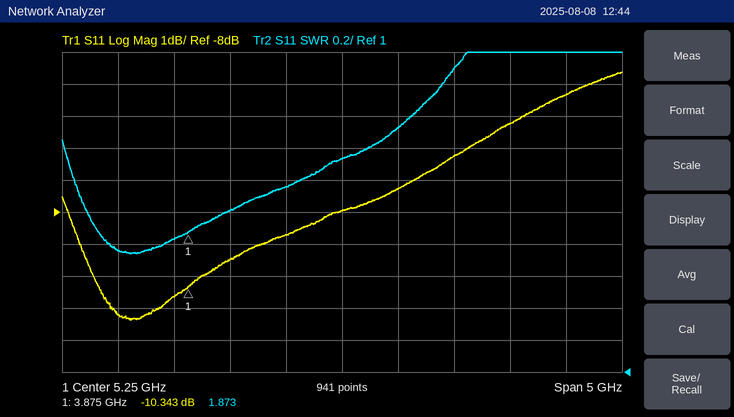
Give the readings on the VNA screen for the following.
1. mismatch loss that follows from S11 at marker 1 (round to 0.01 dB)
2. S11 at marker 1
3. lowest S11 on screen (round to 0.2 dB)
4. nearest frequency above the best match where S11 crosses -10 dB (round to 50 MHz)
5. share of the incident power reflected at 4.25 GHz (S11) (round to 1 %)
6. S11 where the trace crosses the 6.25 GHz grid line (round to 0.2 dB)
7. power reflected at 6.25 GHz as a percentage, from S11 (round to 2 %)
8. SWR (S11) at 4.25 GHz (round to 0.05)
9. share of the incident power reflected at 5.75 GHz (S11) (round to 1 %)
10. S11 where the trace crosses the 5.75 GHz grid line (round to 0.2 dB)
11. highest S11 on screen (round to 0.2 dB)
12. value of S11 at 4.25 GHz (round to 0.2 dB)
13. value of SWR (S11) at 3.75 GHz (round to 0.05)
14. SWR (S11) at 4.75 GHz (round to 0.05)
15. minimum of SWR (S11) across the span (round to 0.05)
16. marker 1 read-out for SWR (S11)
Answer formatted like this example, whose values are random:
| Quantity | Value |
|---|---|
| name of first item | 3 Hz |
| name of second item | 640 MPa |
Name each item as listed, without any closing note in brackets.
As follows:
| Quantity | Value |
|---|---|
| mismatch loss that follows from S11 at marker 1 | 0.42 dB |
| S11 at marker 1 | -10.343 dB |
| lowest S11 on screen | -11.4 dB |
| nearest frequency above the best match where S11 crosses -10 dB | 4.00 GHz |
| share of the incident power reflected at 4.25 GHz (S11) | 11 % |
| S11 where the trace crosses the 6.25 GHz grid line | -6.2 dB |
| power reflected at 6.25 GHz as a percentage, from S11 | 24 % |
| SWR (S11) at 4.25 GHz | 2.00 |
| share of the incident power reflected at 5.75 GHz (S11) | 19 % |
| S11 where the trace crosses the 5.75 GHz grid line | -7.2 dB |
| highest S11 on screen | -3.6 dB |
| value of S11 at 4.25 GHz | -9.4 dB |
| value of SWR (S11) at 3.75 GHz | 1.85 |
| SWR (S11) at 4.75 GHz | 2.15 |
| minimum of SWR (S11) across the span | 1.75 |
| marker 1 read-out for SWR | 1.873 |
